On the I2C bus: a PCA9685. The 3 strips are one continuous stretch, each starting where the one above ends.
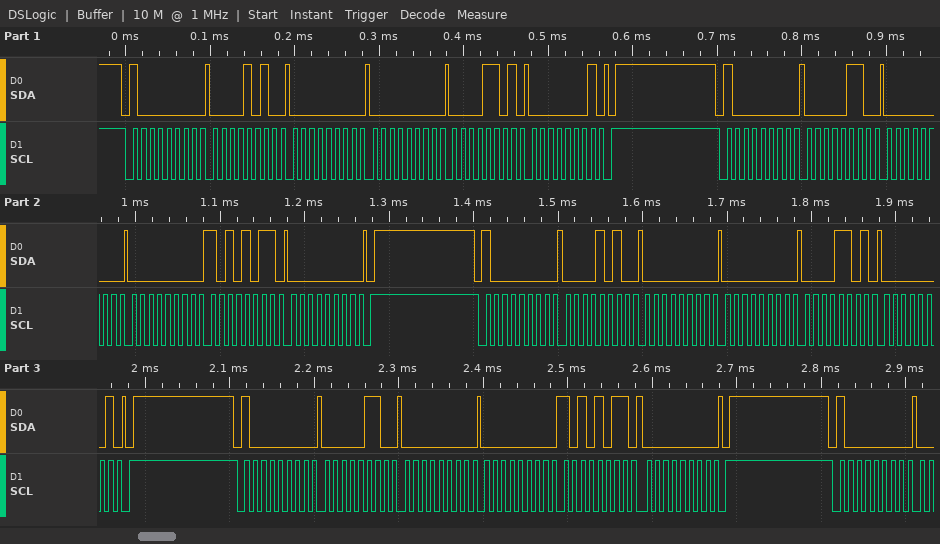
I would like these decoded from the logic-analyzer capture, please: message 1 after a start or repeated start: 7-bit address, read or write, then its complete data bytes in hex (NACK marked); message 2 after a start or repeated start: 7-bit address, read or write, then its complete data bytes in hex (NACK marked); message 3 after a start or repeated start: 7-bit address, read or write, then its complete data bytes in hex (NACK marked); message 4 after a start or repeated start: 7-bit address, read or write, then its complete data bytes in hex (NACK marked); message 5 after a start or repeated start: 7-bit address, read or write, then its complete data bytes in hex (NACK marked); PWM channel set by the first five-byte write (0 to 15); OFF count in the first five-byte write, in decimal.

0x40 write: 0A 00 00 0D 01
0x40 write: 06 00 00 AB 00
0x40 write: 0A 00 00 0D 01
0x40 write: 06 00 00 AB 00
0x40 write
1
269
